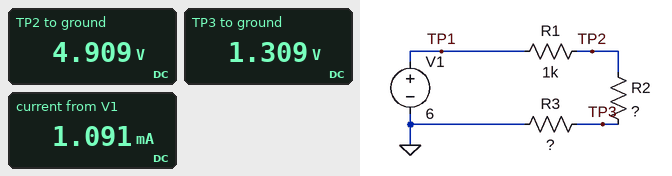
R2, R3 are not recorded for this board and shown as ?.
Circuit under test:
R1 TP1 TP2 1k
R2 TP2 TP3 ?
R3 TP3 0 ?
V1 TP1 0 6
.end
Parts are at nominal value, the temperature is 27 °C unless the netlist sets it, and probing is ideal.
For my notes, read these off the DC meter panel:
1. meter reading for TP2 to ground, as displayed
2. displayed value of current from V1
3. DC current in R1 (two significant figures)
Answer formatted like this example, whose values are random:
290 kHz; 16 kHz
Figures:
4.909 V; 1.091 mA; 1.1 mA
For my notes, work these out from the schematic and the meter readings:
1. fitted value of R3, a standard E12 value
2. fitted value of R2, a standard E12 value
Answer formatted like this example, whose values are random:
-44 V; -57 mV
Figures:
1.2 kΩ; 3.3 kΩ
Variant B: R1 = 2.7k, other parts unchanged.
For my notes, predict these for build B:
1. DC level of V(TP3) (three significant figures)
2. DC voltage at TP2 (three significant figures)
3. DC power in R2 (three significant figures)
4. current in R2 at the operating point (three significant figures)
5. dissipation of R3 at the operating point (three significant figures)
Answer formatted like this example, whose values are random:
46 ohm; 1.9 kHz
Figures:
1.00 V; 3.75 V; 2.29 mW; 833 µA; 833 µW
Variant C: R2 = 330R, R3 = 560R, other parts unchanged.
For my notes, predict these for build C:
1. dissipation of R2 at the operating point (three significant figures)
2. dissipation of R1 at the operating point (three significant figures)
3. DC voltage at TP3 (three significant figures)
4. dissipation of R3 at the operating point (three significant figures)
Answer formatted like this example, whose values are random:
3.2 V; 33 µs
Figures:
3.33 mW; 10.1 mW; 1.78 V; 5.64 mW
